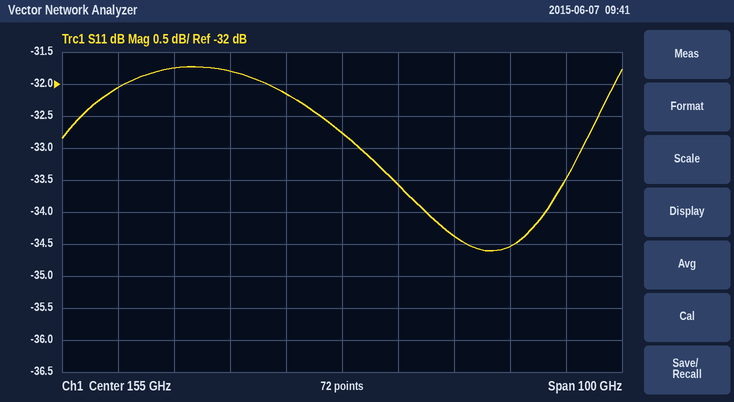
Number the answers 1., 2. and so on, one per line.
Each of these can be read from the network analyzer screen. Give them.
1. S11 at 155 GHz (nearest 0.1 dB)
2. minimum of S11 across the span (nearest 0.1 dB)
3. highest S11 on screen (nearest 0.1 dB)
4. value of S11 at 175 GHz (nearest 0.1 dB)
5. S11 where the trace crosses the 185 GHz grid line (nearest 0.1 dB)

1. -32.8 dB
2. -34.6 dB
3. -31.7 dB
4. -34.4 dB
5. -34.5 dB
